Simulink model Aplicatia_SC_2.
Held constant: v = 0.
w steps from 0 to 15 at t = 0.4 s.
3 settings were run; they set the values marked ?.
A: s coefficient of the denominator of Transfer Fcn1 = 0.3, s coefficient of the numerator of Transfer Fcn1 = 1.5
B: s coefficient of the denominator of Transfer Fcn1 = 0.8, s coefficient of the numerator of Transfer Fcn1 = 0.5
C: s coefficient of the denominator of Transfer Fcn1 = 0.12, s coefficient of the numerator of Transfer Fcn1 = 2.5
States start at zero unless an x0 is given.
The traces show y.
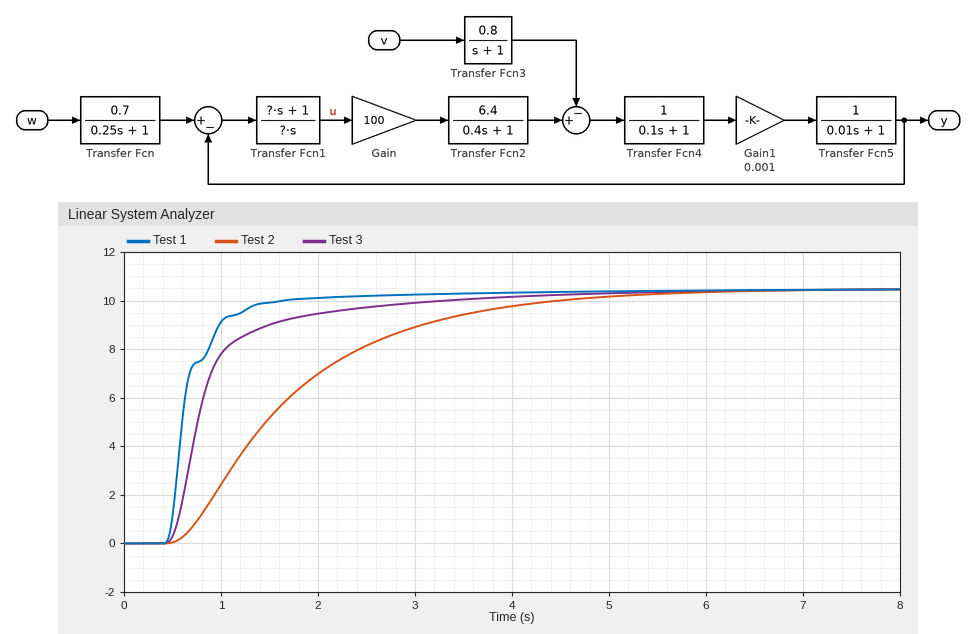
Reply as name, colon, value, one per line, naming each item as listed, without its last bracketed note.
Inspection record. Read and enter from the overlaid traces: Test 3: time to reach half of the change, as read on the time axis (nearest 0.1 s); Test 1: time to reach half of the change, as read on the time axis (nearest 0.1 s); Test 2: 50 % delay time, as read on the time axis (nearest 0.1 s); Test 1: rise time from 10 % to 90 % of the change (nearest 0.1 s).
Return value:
Test 3: time to reach half of the change, as read on the time axis: 0.8 s
Test 1: time to reach half of the change, as read on the time axis: 0.6 s
Test 2: 50 % delay time, as read on the time axis: 1.5 s
Test 1: rise time from 10 % to 90 % of the change: 0.7 s
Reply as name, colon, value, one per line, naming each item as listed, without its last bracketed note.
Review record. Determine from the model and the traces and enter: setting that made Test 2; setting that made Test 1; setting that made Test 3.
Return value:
setting that made Test 2: B
setting that made Test 1: C
setting that made Test 3: A
